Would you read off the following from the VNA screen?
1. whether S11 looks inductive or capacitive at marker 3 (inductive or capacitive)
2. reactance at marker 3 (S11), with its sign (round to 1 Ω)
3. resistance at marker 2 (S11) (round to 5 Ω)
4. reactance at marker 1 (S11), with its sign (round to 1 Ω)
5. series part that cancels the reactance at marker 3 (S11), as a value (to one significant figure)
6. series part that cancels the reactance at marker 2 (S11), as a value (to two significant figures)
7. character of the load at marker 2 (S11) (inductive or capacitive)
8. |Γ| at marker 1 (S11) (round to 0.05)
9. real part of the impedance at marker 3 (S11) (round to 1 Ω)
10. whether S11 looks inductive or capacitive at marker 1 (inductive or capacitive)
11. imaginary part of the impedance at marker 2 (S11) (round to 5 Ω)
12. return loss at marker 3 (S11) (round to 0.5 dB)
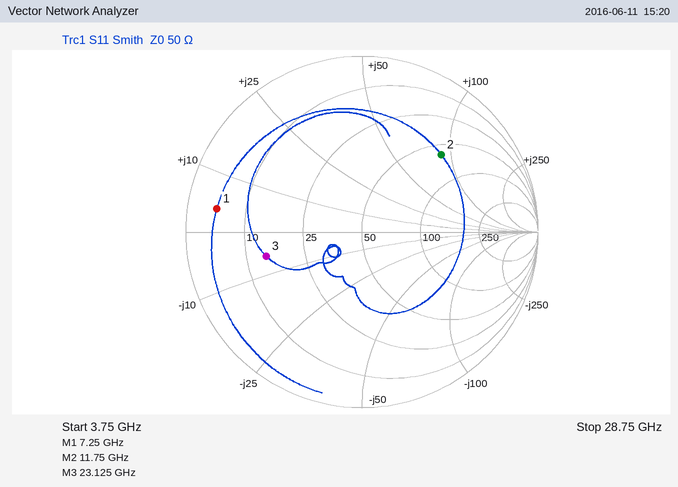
capacitive
-6 Ω
60 Ω
+4 Ω
40 pH
150 fF
inductive
0.85
14 Ω
inductive
+90 Ω
5.0 dB
